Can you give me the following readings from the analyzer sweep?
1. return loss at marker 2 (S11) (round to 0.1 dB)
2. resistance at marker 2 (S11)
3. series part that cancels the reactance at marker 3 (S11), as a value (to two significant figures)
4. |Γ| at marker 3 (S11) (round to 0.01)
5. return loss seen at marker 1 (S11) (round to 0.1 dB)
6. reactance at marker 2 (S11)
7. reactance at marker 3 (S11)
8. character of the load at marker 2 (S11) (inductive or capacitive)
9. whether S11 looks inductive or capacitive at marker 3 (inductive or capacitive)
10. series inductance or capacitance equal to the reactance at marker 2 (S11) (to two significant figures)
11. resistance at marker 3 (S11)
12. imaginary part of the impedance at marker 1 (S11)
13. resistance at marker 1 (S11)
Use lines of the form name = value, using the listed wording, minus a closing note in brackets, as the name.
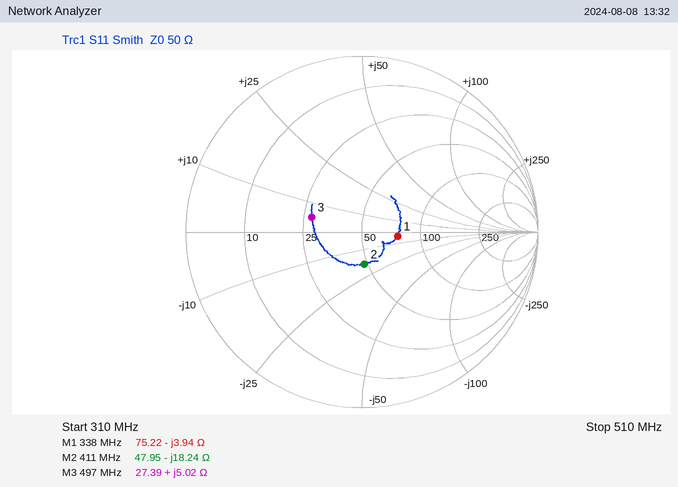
return loss at marker 2 (S11) = 14.7 dB
resistance at marker 2 = 47.95 Ω
series part that cancels the reactance at marker 3 (S11), as a value = 64 pF
|Γ| at marker 3 (S11) = 0.30
return loss seen at marker 1 (S11) = 13.8 dB
reactance at marker 2 = -18.24 Ω
reactance at marker 3 = +5.02 Ω
character of the load at marker 2 (S11) = capacitive
whether S11 looks inductive or capacitive at marker 3 = inductive
series inductance or capacitance equal to the reactance at marker 2 (S11) = 21 pF
resistance at marker 3 = 27.39 Ω
imaginary part of the impedance at marker 1 = -3.94 Ω
resistance at marker 1 = 75.22 Ω
